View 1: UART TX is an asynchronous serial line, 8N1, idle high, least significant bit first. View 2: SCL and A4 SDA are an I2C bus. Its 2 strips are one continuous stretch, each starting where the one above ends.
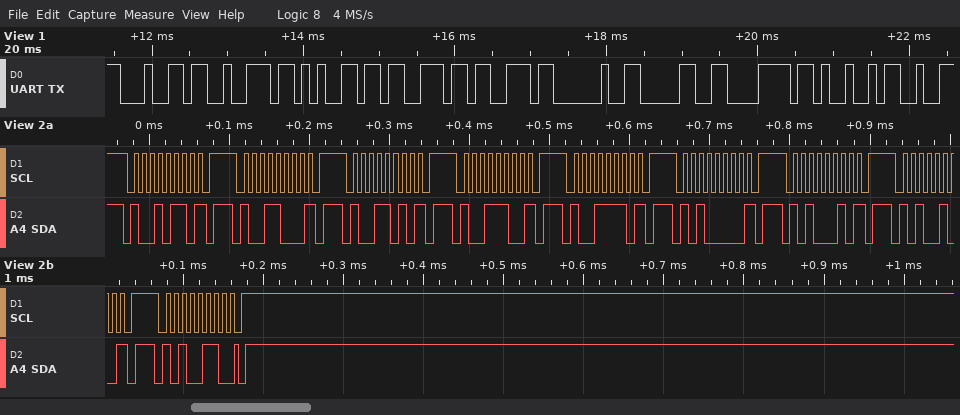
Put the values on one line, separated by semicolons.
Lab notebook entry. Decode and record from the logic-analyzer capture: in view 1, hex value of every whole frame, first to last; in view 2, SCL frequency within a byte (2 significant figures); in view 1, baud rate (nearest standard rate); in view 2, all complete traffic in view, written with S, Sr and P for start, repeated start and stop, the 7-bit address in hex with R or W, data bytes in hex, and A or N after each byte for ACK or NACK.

0x64 0x72 0x65 0x73 0x73 0x20 0x30 0x78 0x49; 100 kHz; 9600 baud; S 4BW N P S 4CW N P S 4DW N P S 4EW N P S 4FW N P S 50W N P S 51W N P S 52W N P S 53W A P
